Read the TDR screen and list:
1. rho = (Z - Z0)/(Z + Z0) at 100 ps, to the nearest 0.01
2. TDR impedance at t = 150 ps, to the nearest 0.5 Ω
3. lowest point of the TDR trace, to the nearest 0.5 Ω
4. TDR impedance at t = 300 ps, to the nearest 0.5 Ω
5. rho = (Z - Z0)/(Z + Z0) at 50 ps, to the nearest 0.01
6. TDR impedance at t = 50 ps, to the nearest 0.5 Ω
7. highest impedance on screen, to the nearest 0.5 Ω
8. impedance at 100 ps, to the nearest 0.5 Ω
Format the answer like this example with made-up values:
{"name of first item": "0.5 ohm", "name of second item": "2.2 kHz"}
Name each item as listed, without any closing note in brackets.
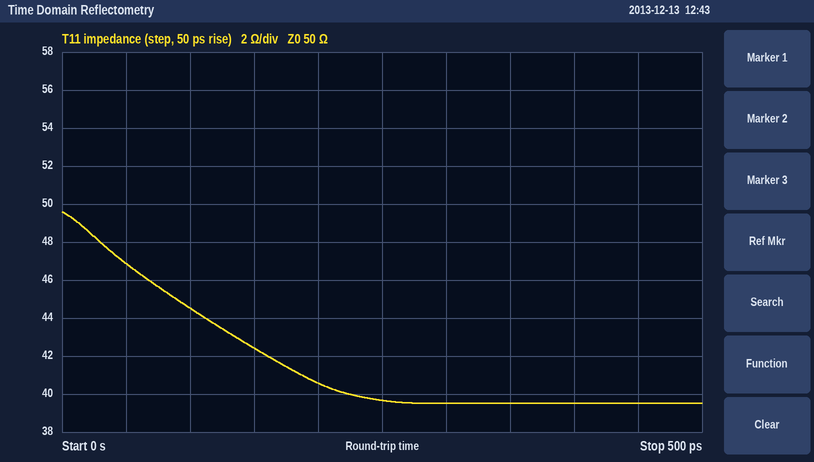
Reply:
{"rho = (Z - Z0)/(Z + Z0) at 100 ps, to the nearest 0.01": "-0.06", "TDR impedance at t = 150 ps, to the nearest 0.5 Ω": "42.5 Ω", "lowest point of the TDR trace, to the nearest 0.5 Ω": "39.5 Ω", "TDR impedance at t = 300 ps, to the nearest 0.5 Ω": "39.5 Ω", "rho = (Z - Z0)/(Z + Z0) at 50 ps, to the nearest 0.01": "-0.03", "TDR impedance at t = 50 ps, to the nearest 0.5 Ω": "47.0 Ω", "highest impedance on screen, to the nearest 0.5 Ω": "49.5 Ω", "impedance at 100 ps, to the nearest 0.5 Ω": "44.5 Ω"}
